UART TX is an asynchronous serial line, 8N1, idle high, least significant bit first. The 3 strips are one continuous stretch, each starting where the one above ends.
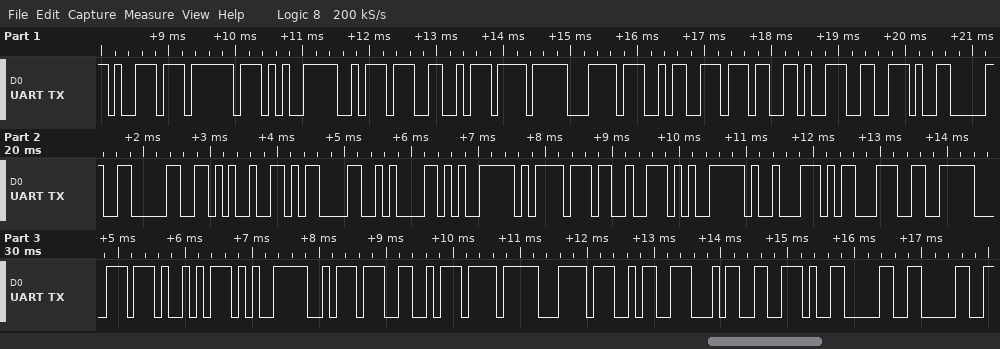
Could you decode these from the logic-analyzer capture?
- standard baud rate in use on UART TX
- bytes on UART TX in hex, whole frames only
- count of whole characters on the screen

9600 baud
B9 BF E5 BA A6 EF BC 9A 37 39 2E 30 30 25 0D 0A E5 BD 93 E5 89 8D E6 B8 A9 E5 BA A6 EF BC 9A 34 2E 30 30
35
